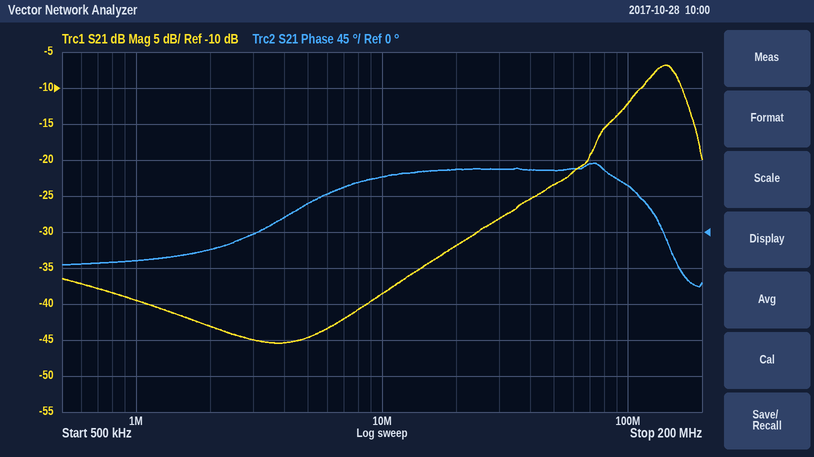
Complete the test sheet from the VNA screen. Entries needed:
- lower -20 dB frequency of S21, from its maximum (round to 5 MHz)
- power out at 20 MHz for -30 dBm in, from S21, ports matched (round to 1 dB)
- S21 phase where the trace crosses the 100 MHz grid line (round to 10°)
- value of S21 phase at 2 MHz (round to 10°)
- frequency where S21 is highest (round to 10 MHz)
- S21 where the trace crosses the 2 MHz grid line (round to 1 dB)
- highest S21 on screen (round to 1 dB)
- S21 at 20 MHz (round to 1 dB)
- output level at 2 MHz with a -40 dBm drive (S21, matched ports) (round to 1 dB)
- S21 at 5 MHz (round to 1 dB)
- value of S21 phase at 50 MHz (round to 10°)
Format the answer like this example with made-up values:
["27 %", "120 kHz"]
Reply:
["35 MHz", "-62 dBm", "60°", "-20°", "140 MHz", "-43 dB", "-7 dB", "-32 dB", "-83 dBm", "-45 dB", "80°"]
